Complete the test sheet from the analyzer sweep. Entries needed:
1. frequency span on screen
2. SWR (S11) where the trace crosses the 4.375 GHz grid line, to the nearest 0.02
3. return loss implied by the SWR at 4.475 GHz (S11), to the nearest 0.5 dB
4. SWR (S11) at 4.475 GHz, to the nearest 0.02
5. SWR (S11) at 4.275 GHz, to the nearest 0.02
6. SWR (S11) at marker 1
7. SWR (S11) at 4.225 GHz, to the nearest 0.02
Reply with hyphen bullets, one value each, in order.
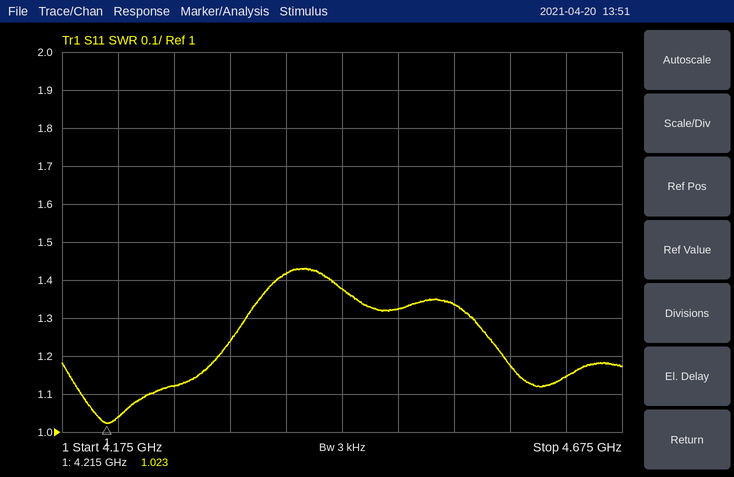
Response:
- 500 MHz
- 1.42
- 17.0 dB
- 1.32
- 1.12
- 1.023
- 1.04
